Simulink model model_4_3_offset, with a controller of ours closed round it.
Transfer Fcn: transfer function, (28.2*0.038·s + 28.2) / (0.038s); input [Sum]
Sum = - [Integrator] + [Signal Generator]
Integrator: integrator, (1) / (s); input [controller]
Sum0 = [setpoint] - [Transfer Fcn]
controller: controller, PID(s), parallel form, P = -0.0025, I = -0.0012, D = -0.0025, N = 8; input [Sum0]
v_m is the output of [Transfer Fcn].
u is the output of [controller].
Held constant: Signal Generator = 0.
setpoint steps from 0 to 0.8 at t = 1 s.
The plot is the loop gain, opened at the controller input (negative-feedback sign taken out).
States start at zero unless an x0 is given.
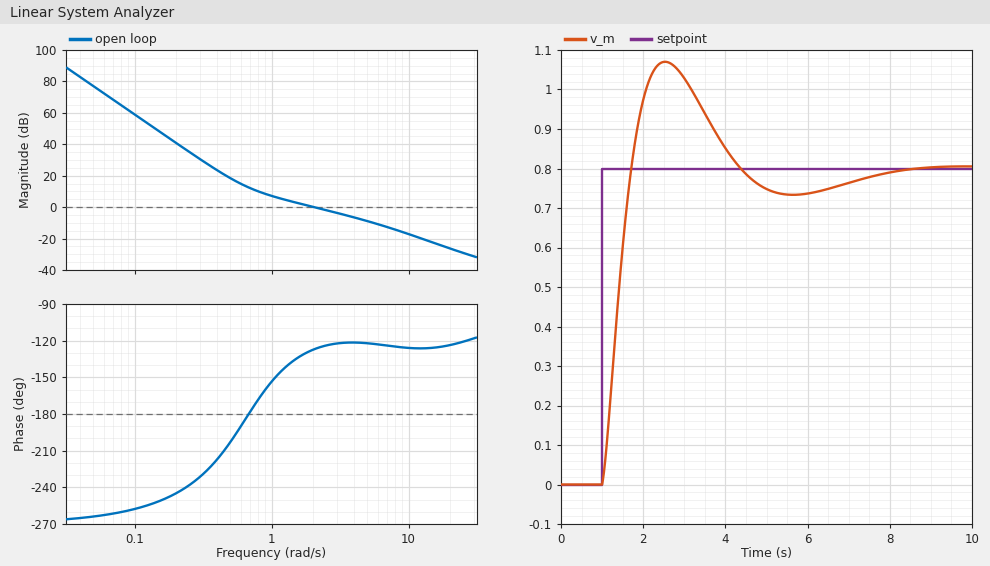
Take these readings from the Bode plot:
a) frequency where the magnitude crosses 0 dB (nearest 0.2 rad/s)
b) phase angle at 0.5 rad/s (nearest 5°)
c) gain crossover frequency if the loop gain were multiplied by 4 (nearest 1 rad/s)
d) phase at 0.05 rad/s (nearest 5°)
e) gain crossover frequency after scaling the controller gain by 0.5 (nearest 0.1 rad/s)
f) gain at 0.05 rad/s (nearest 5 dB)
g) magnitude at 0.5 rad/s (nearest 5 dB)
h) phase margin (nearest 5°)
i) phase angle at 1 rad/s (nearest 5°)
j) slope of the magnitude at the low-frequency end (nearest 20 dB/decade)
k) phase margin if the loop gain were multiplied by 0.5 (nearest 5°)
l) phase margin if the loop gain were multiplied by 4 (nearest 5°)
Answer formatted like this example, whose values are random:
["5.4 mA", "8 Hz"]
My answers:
["2.0 rad/s", "-205°", "7 rad/s", "-265°", "1.1 rad/s", "75 dB", "20 dB", "55°", "-155°", "-60 dB/decade", "30°", "55°"]
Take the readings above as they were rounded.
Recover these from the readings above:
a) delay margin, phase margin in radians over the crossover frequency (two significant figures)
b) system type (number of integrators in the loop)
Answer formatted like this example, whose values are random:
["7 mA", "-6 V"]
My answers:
["0.48 s", "3"]
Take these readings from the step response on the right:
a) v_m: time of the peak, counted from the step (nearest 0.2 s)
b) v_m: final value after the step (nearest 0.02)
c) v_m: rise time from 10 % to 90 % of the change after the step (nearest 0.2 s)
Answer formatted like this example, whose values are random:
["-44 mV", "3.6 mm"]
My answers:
["1.6 s", "0.80", "0.6 s"]
